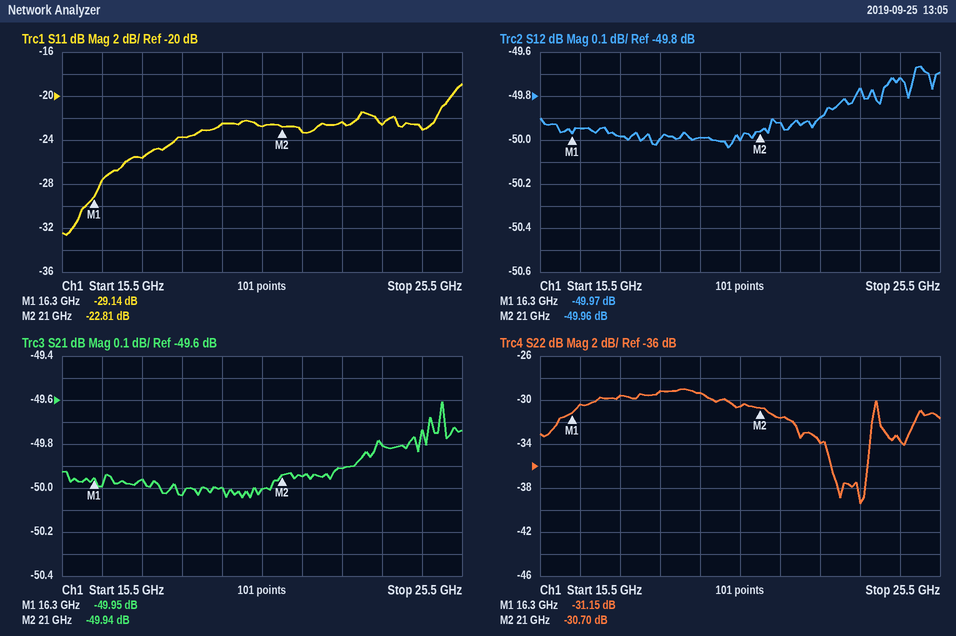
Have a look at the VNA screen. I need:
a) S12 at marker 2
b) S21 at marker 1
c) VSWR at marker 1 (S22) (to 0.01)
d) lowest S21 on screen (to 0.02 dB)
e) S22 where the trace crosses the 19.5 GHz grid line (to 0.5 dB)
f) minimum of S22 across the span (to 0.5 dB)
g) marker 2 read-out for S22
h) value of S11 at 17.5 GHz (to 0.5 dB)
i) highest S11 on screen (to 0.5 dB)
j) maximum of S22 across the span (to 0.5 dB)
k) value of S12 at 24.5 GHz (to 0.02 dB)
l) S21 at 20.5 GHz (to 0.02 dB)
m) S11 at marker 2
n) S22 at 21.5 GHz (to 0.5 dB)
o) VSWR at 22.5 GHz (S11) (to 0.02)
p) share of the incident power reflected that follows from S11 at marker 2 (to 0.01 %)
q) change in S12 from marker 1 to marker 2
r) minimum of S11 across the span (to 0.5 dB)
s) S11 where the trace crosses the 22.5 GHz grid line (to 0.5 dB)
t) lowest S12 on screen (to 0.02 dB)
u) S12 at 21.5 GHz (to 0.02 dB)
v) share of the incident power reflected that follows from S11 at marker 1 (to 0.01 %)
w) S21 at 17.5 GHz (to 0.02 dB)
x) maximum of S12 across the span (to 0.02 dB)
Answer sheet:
-49.96 dB
-49.95 dB
1.06
-50.04 dB
-29.5 dB
-39.5 dB
-30.70 dB
-25.5 dB
-19.0 dB
-29.0 dB
-49.72 dB
-50.00 dB
-22.81 dB
-31.5 dB
1.16
0.52 %
0.01 dB
-32.5 dB
-22.5 dB
-50.04 dB
-49.92 dB
0.12 %
-49.96 dB
-49.66 dB
